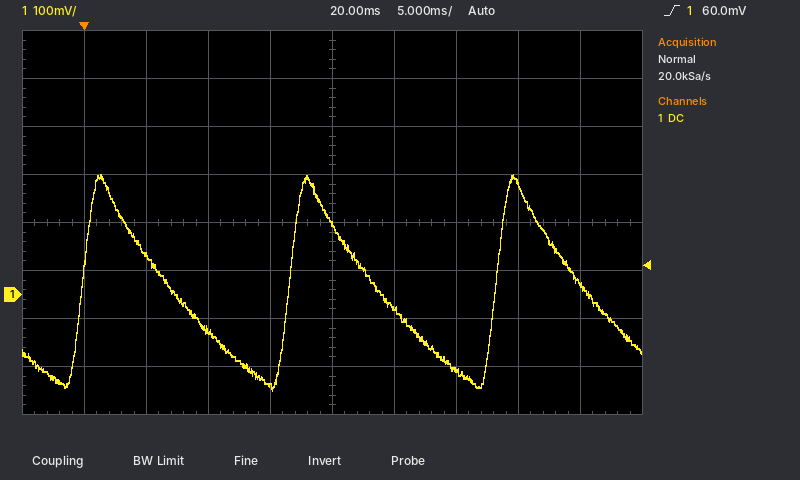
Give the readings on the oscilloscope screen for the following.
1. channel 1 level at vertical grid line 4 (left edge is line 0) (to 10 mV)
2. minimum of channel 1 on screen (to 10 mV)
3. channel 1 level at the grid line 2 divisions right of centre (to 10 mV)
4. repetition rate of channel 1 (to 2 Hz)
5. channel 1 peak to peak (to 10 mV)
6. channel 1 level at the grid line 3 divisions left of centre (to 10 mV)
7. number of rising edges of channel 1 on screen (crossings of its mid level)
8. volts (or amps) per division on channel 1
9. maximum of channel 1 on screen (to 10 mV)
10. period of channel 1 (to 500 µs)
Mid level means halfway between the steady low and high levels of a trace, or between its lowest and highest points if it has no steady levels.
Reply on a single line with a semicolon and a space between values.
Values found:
-190 mV; -200 mV; -160 mV; 60 Hz; 450 mV; 80 mV; 3; 100 mV; 250 mV; 16.5 ms
